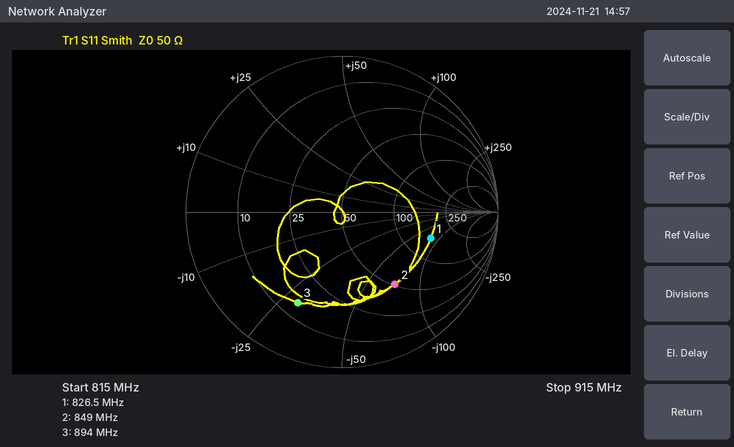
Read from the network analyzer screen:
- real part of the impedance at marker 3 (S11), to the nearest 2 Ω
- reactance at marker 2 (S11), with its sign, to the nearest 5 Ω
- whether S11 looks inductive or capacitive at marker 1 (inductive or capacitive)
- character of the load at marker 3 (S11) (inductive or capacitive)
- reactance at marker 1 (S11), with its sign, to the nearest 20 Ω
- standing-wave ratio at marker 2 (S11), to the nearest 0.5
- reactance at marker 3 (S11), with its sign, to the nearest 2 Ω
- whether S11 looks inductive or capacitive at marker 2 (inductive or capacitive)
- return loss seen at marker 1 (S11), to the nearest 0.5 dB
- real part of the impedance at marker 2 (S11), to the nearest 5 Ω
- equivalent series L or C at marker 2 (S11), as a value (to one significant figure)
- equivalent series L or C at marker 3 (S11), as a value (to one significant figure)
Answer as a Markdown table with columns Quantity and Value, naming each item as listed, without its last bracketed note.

| Quantity | Value |
|---|---|
| real part of the impedance at marker 3 (S11), to the nearest 2 Ω | 14 Ω |
| reactance at marker 2 (S11), with its sign, to the nearest 5 Ω | -70 Ω |
| whether S11 looks inductive or capacitive at marker 1 | capacitive |
| character of the load at marker 3 (S11) | capacitive |
| reactance at marker 1 (S11), with its sign, to the nearest 20 Ω | -80 Ω |
| standing-wave ratio at marker 2 (S11), to the nearest 0.5 | 3.5 |
| reactance at marker 3 (S11), with its sign, to the nearest 2 Ω | -30 Ω |
| whether S11 looks inductive or capacitive at marker 2 | capacitive |
| return loss seen at marker 1 (S11), to the nearest 0.5 dB | 4.5 dB |
| real part of the impedance at marker 2 (S11), to the nearest 5 Ω | 50 Ω |
| equivalent series L or C at marker 2 (S11), as a value | 3 pF |
| equivalent series L or C at marker 3 (S11), as a value | 6 pF |
